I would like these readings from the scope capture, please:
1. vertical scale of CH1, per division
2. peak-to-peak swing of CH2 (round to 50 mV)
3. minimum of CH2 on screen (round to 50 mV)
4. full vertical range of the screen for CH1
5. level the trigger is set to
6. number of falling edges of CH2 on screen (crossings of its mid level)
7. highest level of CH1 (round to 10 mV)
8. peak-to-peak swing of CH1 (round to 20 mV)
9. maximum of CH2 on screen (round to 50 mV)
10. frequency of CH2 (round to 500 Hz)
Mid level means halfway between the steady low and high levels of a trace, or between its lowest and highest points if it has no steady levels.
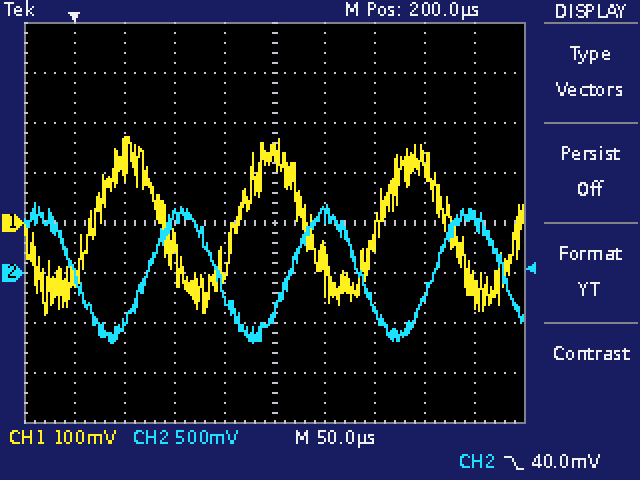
100 mV
1.40 V
-700 mV
800 mV
40.0 mV
4
170 mV
360 mV
700 mV
7.0 kHz
